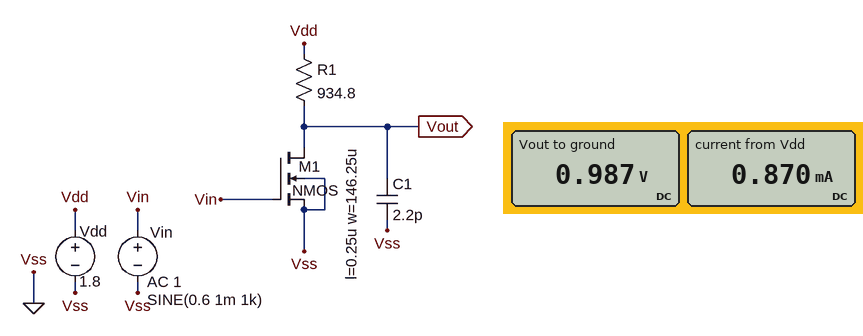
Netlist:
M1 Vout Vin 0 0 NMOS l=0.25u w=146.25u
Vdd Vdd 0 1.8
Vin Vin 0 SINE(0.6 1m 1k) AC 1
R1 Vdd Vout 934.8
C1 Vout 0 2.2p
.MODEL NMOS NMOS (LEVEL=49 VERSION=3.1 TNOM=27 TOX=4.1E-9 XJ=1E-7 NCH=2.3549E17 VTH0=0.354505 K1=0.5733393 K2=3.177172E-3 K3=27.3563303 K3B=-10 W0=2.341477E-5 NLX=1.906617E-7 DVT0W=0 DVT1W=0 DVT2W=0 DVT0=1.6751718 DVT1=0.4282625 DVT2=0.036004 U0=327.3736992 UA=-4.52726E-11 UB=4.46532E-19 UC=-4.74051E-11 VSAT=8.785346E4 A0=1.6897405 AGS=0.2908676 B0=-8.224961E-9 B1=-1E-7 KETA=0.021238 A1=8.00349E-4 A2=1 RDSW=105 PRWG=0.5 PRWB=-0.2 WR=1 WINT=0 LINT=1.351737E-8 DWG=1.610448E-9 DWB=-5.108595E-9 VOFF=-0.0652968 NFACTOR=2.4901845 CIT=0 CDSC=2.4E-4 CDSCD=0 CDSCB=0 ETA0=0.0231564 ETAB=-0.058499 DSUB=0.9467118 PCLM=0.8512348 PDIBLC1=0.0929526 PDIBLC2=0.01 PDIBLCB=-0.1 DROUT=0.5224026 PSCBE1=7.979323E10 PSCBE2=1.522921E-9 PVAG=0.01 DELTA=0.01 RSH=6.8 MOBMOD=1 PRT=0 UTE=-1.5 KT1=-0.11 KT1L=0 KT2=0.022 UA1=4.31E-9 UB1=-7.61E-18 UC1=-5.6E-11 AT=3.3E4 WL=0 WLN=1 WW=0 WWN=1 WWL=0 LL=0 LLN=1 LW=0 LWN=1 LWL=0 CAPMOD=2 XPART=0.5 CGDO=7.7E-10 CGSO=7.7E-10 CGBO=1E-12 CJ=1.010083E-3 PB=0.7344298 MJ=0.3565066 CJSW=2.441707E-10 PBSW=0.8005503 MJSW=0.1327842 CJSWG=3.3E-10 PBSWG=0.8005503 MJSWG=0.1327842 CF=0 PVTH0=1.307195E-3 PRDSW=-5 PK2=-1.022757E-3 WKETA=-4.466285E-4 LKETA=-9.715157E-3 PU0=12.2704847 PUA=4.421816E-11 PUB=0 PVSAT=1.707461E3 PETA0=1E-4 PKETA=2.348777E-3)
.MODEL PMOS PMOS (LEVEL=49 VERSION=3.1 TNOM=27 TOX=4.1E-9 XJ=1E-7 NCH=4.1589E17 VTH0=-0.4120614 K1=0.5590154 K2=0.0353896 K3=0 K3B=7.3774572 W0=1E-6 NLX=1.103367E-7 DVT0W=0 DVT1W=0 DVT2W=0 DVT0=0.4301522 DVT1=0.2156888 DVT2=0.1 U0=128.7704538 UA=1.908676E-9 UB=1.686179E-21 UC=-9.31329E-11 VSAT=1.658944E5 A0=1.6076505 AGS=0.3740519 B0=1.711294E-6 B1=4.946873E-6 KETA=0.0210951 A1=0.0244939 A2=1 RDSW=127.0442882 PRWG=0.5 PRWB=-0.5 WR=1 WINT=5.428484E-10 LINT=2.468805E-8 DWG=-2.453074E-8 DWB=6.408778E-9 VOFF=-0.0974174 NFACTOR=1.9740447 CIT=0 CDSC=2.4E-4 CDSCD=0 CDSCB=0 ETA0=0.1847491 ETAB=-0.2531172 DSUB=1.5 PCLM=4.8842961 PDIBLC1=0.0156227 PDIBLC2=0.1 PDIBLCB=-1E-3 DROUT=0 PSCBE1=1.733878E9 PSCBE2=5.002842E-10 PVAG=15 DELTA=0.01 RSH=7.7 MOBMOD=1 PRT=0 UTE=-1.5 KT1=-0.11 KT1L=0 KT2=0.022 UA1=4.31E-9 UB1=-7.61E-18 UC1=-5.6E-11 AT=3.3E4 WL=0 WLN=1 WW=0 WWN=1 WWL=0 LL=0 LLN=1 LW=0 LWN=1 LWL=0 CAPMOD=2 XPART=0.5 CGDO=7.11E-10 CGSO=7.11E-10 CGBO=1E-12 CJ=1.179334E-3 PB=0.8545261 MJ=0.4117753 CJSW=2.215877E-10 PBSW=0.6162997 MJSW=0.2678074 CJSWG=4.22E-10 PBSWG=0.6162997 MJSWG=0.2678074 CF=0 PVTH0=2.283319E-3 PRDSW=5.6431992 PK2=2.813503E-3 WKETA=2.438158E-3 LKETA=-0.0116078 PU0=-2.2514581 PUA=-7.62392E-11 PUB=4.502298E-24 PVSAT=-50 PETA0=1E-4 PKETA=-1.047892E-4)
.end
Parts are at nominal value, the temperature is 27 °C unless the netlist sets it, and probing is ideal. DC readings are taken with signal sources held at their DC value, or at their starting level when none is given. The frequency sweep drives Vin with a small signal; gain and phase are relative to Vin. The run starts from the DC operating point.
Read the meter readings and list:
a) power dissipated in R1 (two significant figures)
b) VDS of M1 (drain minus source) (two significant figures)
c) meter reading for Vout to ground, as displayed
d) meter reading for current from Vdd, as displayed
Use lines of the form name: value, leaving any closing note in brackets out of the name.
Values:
power dissipated in R1: 710 µW
VDS of M1 (drain minus source): 990 mV
meter reading for Vout to ground, as displayed: 0.987 V
meter reading for current from Vdd, as displayed: 0.870 mA
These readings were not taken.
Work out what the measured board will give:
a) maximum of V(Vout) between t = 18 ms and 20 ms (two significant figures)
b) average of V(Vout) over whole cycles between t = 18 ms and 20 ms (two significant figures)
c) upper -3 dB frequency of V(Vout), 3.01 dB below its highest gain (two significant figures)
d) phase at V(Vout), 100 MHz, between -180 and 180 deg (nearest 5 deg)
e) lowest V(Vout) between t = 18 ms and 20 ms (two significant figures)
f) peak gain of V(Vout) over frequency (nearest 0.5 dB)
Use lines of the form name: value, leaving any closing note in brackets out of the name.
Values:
maximum of V(Vout) between t = 18 ms and 20 ms: 1.0 V
average of V(Vout) over whole cycles between t = 18 ms and 20 ms: 990 mV
upper -3 dB frequency of V(Vout), 3.01 dB below its highest gain: 84 MHz
phase at V(Vout), 100 MHz, between -180 and 180 deg: 130 deg
lowest V(Vout) between t = 18 ms and 20 ms: 980 mV
peak gain of V(Vout) over frequency: 20.5 dB
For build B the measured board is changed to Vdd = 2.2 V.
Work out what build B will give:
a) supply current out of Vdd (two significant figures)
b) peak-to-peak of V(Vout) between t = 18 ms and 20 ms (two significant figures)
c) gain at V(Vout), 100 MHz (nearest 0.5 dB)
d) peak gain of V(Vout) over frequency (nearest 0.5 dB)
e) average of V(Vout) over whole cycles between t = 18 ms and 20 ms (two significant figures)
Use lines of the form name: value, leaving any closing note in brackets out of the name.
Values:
supply current out of Vdd: 930 µA
peak-to-peak of V(Vout) between t = 18 ms and 20 ms: 22 mV
gain at V(Vout), 100 MHz: 17.0 dB
peak gain of V(Vout) over frequency: 21.0 dB
average of V(Vout) over whole cycles between t = 18 ms and 20 ms: 1.3 V
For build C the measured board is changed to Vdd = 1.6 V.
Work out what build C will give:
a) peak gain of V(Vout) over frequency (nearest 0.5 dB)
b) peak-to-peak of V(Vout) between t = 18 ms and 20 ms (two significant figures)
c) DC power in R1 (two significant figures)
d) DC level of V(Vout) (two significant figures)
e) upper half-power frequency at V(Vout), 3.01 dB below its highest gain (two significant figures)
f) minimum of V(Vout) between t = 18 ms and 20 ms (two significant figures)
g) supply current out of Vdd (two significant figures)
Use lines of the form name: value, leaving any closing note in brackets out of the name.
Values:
peak gain of V(Vout) over frequency: 20.0 dB
peak-to-peak of V(Vout) between t = 18 ms and 20 ms: 20 mV
DC power in R1: 660 µW
DC level of V(Vout): 810 mV
upper half-power frequency at V(Vout), 3.01 dB below its highest gain: 84 MHz
minimum of V(Vout) between t = 18 ms and 20 ms: 800 mV
supply current out of Vdd: 840 µA
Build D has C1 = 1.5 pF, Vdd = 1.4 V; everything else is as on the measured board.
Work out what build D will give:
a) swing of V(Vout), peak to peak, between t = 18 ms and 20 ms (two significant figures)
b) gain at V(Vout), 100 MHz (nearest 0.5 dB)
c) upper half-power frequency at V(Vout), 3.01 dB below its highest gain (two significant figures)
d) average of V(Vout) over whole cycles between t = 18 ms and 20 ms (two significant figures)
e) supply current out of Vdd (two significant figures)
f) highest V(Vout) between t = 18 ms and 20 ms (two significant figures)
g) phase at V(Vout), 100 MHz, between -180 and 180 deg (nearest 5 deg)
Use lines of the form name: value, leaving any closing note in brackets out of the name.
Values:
swing of V(Vout), peak to peak, between t = 18 ms and 20 ms: 20 mV
gain at V(Vout), 100 MHz: 17.5 dB
upper half-power frequency at V(Vout), 3.01 dB below its highest gain: 120 MHz
average of V(Vout) over whole cycles between t = 18 ms and 20 ms: 640 mV
supply current out of Vdd: 810 µA
highest V(Vout) between t = 18 ms and 20 ms: 650 mV
phase at V(Vout), 100 MHz, between -180 and 180 deg: 140 deg
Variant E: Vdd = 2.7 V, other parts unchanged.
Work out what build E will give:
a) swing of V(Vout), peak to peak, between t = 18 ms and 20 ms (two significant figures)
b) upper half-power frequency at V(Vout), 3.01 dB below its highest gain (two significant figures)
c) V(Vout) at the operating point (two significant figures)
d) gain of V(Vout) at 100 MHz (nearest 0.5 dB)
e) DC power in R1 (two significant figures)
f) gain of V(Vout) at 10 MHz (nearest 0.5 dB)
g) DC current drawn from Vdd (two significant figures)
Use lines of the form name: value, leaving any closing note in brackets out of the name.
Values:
swing of V(Vout), peak to peak, between t = 18 ms and 20 ms: 23 mV
upper half-power frequency at V(Vout), 3.01 dB below its highest gain: 83 MHz
V(Vout) at the operating point: 1.8 V
gain of V(Vout) at 100 MHz: 17.5 dB
DC power in R1: 930 µW
gain of V(Vout) at 10 MHz: 21.0 dB
DC current drawn from Vdd: 1.0 mA
